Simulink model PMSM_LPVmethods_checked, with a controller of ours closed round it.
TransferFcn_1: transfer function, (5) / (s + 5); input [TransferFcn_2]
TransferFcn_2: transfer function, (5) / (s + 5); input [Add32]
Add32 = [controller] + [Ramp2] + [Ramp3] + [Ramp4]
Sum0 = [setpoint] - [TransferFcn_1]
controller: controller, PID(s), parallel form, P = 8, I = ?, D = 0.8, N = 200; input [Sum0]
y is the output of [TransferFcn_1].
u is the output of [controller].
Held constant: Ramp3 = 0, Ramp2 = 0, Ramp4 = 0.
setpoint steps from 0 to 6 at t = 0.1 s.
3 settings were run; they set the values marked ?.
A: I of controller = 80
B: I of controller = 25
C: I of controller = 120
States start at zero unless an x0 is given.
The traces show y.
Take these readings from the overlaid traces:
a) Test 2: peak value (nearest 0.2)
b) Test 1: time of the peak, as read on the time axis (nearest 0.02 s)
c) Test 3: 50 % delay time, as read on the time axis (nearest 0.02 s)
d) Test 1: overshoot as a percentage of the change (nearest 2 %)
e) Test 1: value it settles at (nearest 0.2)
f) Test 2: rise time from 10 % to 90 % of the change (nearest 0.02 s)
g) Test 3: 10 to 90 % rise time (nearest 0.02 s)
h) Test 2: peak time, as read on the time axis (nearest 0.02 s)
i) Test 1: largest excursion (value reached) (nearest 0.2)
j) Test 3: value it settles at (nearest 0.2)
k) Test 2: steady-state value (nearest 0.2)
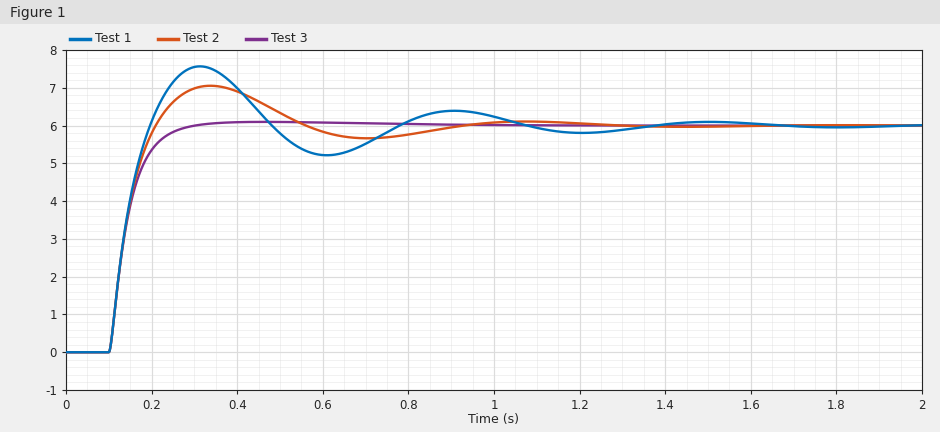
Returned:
7.0
0.32 s
0.14 s
26 %
6.0
0.08 s
0.10 s
0.34 s
7.6
6.0
6.0
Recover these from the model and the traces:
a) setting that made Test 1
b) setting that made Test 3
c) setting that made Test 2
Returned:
C
B
A
